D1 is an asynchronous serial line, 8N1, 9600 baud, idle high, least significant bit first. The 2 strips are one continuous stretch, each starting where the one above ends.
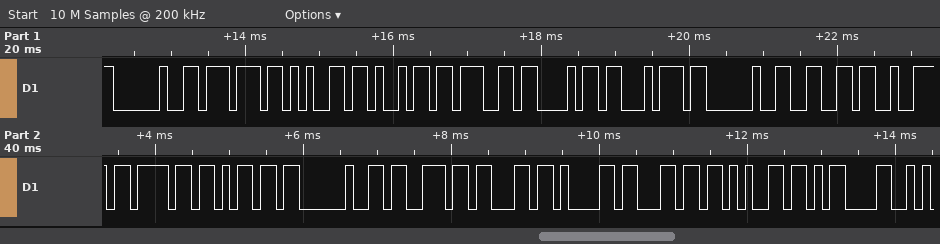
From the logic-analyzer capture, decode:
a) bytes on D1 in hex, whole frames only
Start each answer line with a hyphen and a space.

- 20 77 65 69 67 68 74 20 66 72 6F 6D 20 73 63 61 6C 65 0D
